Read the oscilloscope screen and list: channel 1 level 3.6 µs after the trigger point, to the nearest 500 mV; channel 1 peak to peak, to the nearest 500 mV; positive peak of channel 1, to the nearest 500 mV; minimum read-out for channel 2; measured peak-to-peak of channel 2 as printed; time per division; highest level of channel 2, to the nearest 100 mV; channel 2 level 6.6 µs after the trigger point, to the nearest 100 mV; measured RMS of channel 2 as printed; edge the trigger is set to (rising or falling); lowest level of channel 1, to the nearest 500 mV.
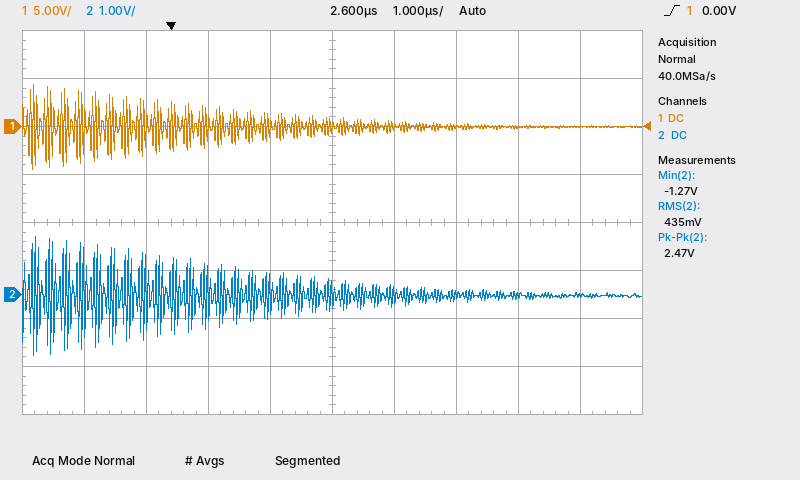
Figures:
0.0 V
9.0 V
4.5 V
-1.27 V
2.47 V
1 µs
1.2 V
0.0 V
435 mV
rising
-4.5 V
